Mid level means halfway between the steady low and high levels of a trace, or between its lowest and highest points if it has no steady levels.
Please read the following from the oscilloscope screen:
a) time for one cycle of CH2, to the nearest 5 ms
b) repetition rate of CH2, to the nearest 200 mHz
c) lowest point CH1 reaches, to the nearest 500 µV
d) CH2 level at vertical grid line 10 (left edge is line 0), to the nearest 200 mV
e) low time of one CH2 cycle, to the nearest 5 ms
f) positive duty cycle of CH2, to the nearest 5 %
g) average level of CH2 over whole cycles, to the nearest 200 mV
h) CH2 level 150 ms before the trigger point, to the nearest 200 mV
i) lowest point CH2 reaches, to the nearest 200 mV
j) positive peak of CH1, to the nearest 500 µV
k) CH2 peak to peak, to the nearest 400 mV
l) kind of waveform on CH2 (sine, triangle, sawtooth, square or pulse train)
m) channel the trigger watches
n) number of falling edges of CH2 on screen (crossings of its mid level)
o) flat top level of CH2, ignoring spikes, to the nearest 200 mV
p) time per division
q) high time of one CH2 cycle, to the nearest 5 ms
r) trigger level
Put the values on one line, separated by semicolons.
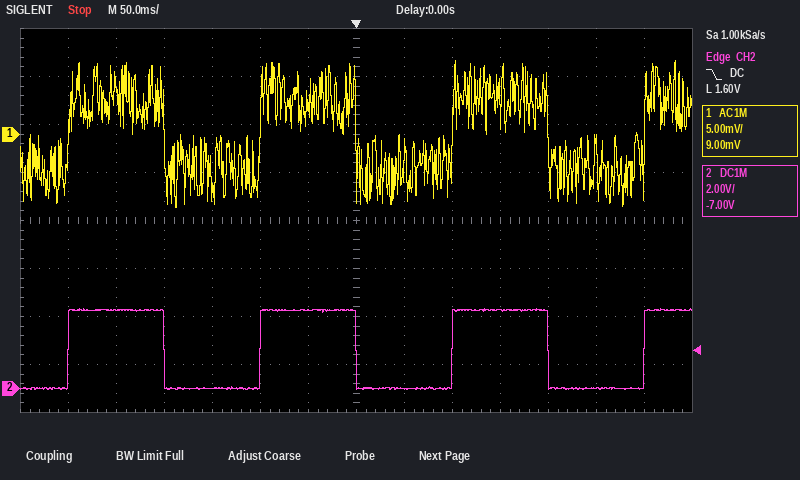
200 ms; 5.0 Hz; -7.5 mV; 3.2 V; 100 ms; 50 %; 1.6 V; 0.0 V; 0.0 V; 7.5 mV; 3.2 V; square; CH2; 3; 3.2 V; 50 ms; 100 ms; 1.60 V
